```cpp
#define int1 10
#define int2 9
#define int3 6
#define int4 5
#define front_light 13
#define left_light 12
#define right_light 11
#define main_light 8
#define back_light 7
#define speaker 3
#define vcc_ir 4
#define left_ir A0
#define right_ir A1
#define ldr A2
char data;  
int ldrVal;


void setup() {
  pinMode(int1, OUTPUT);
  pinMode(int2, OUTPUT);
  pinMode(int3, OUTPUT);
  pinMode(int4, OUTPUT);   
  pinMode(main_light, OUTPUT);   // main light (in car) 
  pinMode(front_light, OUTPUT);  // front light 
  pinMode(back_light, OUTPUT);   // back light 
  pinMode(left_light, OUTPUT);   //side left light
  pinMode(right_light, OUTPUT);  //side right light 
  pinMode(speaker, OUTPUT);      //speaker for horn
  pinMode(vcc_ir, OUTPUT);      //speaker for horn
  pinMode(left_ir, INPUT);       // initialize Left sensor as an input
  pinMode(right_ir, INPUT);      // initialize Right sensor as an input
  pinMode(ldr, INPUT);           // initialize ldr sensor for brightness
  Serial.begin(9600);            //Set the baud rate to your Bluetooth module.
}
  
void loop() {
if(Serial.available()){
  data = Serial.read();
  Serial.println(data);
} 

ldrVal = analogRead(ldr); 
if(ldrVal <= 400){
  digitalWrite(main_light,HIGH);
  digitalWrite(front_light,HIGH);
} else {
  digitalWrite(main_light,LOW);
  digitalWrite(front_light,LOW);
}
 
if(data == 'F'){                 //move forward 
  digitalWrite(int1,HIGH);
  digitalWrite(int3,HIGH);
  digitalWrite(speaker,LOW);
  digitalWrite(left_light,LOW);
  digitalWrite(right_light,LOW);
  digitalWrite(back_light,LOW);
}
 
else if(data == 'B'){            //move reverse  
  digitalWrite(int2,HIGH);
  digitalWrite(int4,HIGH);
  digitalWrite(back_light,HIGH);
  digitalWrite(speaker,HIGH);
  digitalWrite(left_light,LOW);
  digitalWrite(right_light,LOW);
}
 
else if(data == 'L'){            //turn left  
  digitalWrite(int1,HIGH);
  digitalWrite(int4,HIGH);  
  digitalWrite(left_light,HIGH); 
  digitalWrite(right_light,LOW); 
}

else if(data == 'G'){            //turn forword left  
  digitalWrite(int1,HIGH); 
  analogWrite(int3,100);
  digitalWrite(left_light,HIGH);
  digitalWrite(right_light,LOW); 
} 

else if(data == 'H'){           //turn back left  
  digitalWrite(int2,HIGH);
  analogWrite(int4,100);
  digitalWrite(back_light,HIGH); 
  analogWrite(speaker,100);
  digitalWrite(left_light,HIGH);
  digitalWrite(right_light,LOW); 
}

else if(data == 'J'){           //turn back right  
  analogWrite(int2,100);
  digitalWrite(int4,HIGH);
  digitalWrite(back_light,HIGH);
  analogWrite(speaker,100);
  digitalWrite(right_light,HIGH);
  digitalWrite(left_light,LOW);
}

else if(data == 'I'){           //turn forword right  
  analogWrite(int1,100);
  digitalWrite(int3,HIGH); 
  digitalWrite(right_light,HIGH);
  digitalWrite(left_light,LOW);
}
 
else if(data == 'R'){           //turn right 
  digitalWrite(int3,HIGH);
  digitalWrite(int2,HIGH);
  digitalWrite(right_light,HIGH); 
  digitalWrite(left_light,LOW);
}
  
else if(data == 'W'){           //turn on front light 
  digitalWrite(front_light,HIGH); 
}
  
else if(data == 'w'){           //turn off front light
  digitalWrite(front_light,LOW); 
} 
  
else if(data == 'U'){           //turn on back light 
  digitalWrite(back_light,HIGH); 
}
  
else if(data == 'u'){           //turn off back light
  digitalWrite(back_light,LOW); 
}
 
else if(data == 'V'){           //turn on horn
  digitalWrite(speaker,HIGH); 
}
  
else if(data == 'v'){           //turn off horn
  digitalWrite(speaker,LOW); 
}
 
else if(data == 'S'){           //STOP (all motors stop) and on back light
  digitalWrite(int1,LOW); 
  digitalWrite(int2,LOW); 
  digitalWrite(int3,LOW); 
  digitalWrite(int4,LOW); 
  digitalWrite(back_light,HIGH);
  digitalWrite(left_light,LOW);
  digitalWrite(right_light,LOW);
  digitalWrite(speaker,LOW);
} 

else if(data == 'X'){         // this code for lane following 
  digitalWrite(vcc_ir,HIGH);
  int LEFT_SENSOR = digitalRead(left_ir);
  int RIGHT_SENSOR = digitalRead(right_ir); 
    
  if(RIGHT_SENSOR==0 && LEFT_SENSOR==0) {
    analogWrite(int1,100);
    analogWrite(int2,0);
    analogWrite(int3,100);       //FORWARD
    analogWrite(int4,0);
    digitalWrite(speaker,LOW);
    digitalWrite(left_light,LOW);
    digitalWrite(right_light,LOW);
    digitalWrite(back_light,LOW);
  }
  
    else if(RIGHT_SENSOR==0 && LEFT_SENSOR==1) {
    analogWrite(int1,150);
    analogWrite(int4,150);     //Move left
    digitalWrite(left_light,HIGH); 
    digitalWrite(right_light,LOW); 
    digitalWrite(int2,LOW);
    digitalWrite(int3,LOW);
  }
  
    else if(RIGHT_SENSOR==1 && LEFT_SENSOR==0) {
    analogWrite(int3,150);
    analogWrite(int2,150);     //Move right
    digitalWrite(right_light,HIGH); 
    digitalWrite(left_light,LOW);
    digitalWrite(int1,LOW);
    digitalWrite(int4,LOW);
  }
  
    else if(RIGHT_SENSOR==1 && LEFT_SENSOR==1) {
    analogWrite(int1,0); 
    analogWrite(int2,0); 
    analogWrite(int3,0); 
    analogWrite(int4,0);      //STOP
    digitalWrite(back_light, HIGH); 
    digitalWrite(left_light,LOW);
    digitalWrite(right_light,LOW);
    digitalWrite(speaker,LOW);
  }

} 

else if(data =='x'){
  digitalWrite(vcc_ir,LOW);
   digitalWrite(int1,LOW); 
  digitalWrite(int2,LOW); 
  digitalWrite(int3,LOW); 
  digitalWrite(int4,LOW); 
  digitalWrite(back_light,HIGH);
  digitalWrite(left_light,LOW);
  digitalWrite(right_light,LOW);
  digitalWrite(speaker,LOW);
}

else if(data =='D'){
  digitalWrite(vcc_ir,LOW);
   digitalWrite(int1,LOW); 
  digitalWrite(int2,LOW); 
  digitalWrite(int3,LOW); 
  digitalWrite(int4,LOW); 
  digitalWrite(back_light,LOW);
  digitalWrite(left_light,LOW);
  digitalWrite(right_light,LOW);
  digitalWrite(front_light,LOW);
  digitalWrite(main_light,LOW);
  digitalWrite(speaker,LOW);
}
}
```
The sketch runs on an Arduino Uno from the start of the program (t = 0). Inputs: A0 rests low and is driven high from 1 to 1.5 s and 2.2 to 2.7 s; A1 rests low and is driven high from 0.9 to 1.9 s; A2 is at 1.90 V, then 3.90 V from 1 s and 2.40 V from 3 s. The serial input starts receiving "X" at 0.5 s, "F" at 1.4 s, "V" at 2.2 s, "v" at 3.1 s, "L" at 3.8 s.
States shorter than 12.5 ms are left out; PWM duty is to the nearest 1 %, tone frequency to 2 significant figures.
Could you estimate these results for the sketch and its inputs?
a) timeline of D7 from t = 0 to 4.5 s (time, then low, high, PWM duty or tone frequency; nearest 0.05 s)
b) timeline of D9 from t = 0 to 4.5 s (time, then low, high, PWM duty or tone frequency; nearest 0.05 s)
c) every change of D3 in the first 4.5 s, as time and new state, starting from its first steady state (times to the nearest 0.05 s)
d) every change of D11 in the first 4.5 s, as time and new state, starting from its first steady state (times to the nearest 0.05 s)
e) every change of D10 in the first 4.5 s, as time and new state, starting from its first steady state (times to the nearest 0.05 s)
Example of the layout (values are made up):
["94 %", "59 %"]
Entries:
["0 s low; 1 s high; 1.4 s low", "0 s low; 0.9 s PWM 59 %; 1 s low", "0 s low; 2.2 s high; 3.1 s low", "0 s low; 0.9 s high; 1 s low", "0 s low; 0.5 s PWM 39 %; 0.9 s low; 1.4 s high"]
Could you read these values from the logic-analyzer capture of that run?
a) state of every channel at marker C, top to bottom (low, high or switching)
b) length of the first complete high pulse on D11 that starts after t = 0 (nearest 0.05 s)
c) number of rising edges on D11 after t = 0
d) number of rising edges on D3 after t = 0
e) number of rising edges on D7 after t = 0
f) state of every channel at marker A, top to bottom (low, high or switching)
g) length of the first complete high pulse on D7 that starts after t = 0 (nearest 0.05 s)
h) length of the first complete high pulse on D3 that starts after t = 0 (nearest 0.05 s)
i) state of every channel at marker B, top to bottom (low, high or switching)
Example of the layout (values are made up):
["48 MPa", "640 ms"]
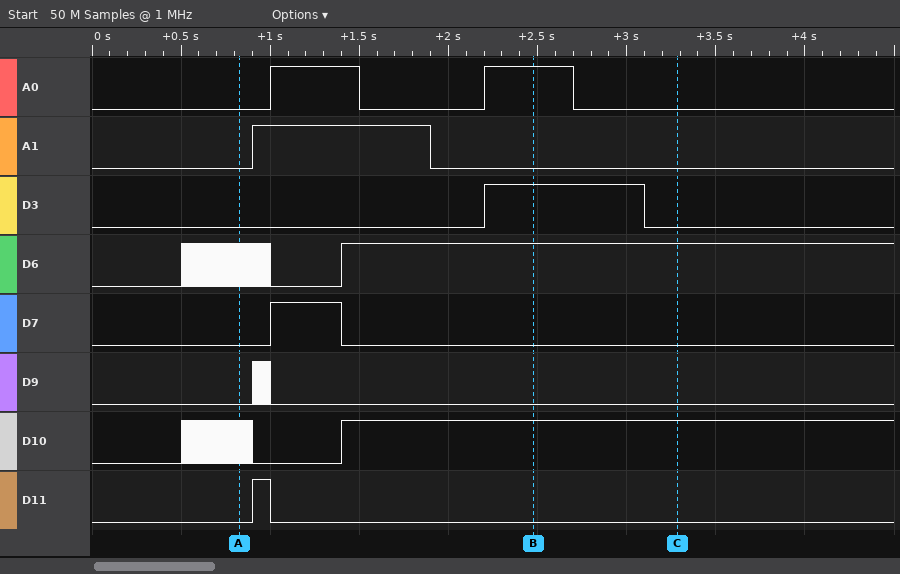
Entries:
["A0 low, A1 low, D3 low, D6 high, D7 low, D9 low, D10 high, D11 low", "0.10 s", "1", "1", "1", "A0 low, A1 low, D3 low, D6 switching, D7 low, D9 low, D10 switching, D11 low", "0.40 s", "0.90 s", "A0 high, A1 low, D3 high, D6 high, D7 low, D9 low, D10 high, D11 low"]
